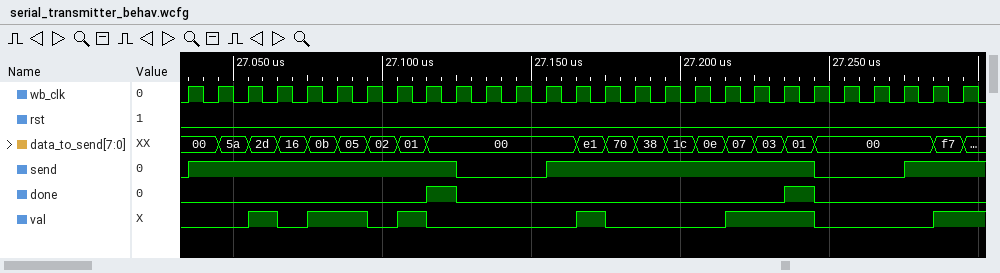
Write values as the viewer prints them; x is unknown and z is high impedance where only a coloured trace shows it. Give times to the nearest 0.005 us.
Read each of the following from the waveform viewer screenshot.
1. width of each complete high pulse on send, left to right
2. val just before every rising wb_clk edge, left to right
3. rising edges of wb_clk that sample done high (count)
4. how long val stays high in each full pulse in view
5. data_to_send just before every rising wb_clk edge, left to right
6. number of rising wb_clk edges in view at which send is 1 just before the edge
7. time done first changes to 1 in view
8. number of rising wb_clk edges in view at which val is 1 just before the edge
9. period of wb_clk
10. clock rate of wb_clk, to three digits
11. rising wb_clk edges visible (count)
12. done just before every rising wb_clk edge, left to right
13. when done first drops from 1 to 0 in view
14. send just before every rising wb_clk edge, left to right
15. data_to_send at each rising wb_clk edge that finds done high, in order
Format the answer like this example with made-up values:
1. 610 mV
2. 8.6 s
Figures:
1. 0.09 us, 0.09 us
2. 0 0 0 1 0 1 1 0 1 0 0 0 0 0 1 0 0 0 0 1 1 1 0 0 0 0 1
3. 2
4. 0.01 us, 0.02 us, 0.01 us, 0.01 us, 0.03 us
5. 00, 00, 5a, 2d, 16, 0b, 05, 02, 01, 00, 00, 00, 00, 00, e1, 70, 38, 1c, 0e, 07, 03, 01, 00, 00, 00, 00, f7
6. 20
7. 27.115 us
8. 9
9. 0.01 us
10. 100 MHz
11. 27
12. 0 0 0 0 0 0 0 0 0 1 0 0 0 0 0 0 0 0 0 0 0 1 0 0 0 0 0
13. 27.125 us
14. 0 1 1 1 1 1 1 1 1 1 0 0 0 1 1 1 1 1 1 1 1 1 0 0 0 1 1
15. 00, 01
